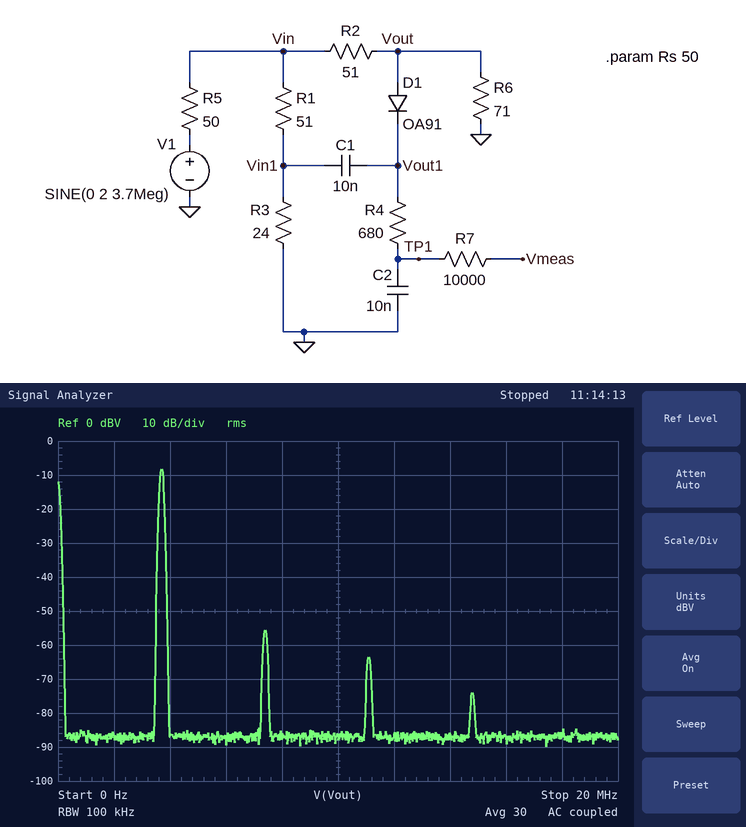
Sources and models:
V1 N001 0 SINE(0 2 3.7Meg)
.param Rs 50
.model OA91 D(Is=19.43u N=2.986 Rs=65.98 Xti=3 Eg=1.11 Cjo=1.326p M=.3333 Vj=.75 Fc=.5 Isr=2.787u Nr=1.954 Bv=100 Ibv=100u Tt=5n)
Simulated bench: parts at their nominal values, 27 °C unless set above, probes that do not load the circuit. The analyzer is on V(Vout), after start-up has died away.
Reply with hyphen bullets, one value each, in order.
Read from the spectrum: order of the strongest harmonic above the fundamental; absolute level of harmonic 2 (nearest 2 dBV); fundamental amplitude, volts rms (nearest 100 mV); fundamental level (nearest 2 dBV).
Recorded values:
- 2
- -56 dBV
- 400 mV
- -8 dBV
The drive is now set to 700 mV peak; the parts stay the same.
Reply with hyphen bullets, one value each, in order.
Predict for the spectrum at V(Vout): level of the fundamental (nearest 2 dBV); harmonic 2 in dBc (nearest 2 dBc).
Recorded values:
- -18 dBV
- -56 dBc
